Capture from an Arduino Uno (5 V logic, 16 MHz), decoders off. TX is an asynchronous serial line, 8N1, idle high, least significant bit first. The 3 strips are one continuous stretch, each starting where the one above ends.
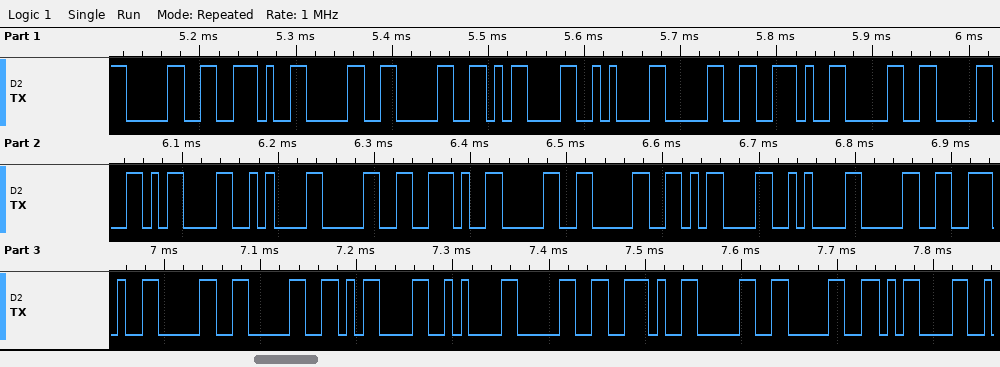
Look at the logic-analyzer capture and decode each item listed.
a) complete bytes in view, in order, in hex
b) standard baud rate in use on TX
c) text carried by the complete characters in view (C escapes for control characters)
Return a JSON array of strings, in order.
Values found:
["30 2E 30 30 0D 0A 30 2E 30 30 0D 0A 30 2E 30 30 0D 0A 30 2E 30 30 0D 0A 30 2E 30 30 0D", "115200 baud", "\"0.00\\r\\n0.00\\r\\n0.00\\r\\n0.00\\r\\n0.00\\r\""]
